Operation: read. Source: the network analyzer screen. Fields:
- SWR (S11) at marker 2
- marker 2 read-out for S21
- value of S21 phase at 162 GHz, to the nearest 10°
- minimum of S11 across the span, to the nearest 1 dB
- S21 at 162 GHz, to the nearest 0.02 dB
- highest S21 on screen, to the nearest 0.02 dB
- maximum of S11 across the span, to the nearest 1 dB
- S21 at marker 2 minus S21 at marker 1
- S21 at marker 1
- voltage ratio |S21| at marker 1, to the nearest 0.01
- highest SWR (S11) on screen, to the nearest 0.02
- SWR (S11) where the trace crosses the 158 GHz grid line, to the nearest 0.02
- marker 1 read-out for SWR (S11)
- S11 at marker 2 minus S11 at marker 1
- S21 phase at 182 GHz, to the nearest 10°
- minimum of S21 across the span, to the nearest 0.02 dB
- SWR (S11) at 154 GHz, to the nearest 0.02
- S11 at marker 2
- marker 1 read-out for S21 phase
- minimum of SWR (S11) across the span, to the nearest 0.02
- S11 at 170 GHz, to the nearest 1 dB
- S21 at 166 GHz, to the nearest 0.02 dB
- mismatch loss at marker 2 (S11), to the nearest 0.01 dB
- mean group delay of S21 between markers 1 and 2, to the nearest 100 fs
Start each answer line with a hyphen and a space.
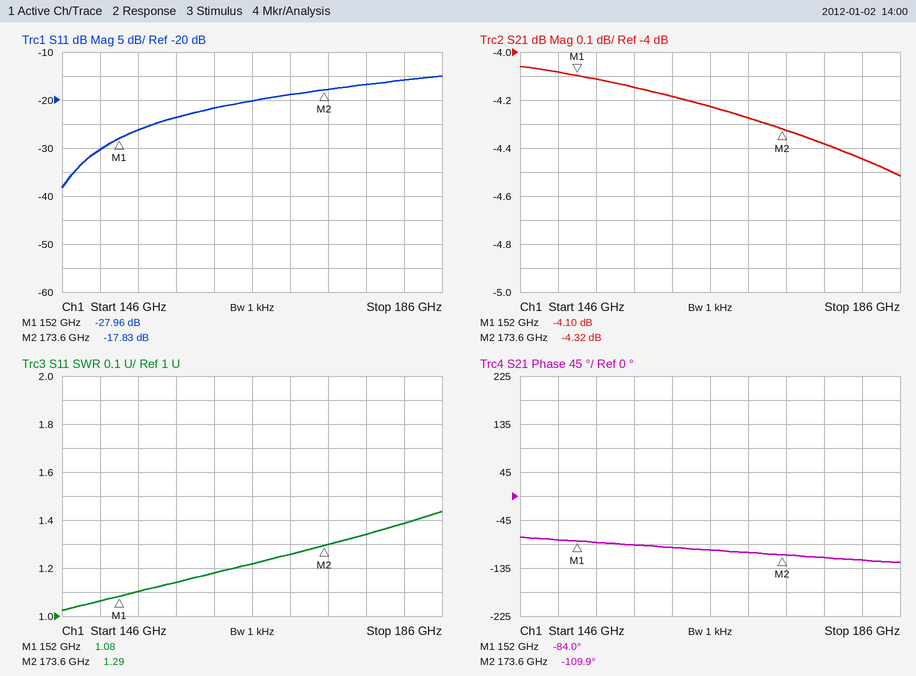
- 1.29
- -4.32 dB
- -100°
- -38 dB
- -4.18 dB
- -4.06 dB
- -15 dB
- -0.22 dB
- -4.10 dB
- 0.62
- 1.44
- 1.14
- 1.08
- 10.13 dB
- -120°
- -4.52 dB
- 1.10
- -17.83 dB
- -84.0°
- 1.02
- -19 dB
- -4.22 dB
- 0.07 dB
- 3.3 ps
